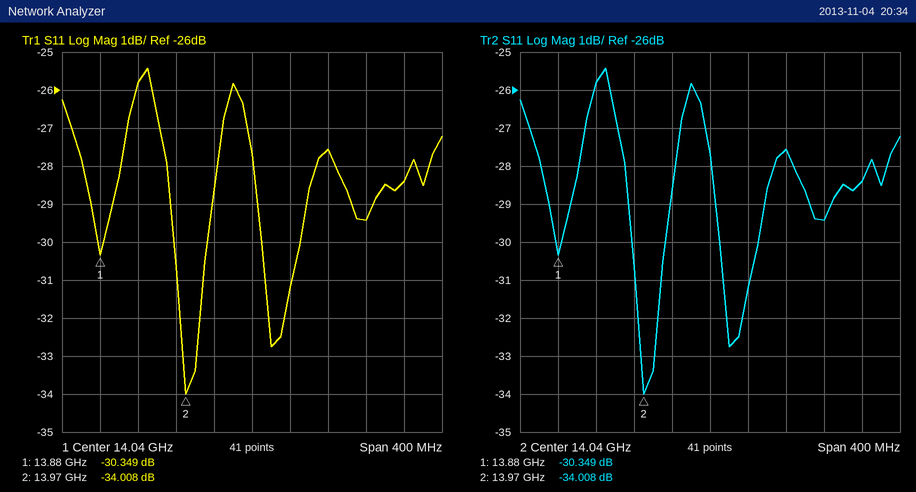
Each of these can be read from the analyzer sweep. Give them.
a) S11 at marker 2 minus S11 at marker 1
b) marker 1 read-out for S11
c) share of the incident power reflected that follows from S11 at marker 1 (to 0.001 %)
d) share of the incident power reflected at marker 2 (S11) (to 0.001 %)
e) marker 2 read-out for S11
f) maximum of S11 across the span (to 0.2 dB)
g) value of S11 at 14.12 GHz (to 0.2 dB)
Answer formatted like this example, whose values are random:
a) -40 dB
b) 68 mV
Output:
a) -3.659 dB
b) -30.349 dB
c) 0.092 %
d) 0.040 %
e) -34.008 dB
f) -25.4 dB
g) -27.6 dB
